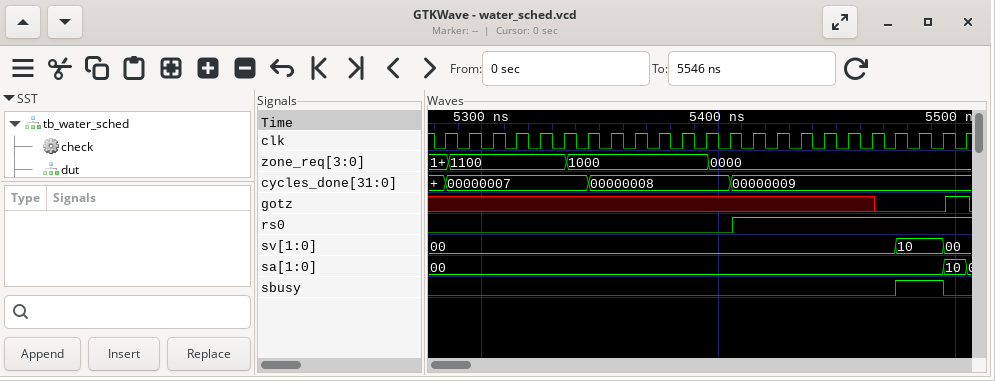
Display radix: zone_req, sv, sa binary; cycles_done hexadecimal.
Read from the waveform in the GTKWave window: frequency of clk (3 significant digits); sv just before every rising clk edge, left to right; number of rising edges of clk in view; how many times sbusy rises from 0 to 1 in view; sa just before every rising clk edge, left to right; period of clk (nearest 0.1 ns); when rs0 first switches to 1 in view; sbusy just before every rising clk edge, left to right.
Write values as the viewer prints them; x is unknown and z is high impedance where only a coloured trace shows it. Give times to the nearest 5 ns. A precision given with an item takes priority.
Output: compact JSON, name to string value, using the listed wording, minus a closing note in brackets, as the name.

{"frequency of clk": "100 MHz", "sv just before every rising clk edge, left to right": "00, 00, 00, 00, 00, 00, 00, 00, 00, 00, 00, 00, 00, 00, 00, 00, 00, 00, 00, 00, 10, 10, 00", "number of rising edges of clk in view": "23", "how many times sbusy rises from 0 to 1 in view": "1", "sa just before every rising clk edge, left to right": "00, 00, 00, 00, 00, 00, 00, 00, 00, 00, 00, 00, 00, 00, 00, 00, 00, 00, 00, 00, 00, 00, 10", "period of clk": "10 ns", "when rs0 first switches to 1 in view": "5405 ns", "sbusy just before every rising clk edge, left to right": "0 0 0 0 0 0 0 0 0 0 0 0 0 0 0 0 0 0 0 0 1 1 0"}
